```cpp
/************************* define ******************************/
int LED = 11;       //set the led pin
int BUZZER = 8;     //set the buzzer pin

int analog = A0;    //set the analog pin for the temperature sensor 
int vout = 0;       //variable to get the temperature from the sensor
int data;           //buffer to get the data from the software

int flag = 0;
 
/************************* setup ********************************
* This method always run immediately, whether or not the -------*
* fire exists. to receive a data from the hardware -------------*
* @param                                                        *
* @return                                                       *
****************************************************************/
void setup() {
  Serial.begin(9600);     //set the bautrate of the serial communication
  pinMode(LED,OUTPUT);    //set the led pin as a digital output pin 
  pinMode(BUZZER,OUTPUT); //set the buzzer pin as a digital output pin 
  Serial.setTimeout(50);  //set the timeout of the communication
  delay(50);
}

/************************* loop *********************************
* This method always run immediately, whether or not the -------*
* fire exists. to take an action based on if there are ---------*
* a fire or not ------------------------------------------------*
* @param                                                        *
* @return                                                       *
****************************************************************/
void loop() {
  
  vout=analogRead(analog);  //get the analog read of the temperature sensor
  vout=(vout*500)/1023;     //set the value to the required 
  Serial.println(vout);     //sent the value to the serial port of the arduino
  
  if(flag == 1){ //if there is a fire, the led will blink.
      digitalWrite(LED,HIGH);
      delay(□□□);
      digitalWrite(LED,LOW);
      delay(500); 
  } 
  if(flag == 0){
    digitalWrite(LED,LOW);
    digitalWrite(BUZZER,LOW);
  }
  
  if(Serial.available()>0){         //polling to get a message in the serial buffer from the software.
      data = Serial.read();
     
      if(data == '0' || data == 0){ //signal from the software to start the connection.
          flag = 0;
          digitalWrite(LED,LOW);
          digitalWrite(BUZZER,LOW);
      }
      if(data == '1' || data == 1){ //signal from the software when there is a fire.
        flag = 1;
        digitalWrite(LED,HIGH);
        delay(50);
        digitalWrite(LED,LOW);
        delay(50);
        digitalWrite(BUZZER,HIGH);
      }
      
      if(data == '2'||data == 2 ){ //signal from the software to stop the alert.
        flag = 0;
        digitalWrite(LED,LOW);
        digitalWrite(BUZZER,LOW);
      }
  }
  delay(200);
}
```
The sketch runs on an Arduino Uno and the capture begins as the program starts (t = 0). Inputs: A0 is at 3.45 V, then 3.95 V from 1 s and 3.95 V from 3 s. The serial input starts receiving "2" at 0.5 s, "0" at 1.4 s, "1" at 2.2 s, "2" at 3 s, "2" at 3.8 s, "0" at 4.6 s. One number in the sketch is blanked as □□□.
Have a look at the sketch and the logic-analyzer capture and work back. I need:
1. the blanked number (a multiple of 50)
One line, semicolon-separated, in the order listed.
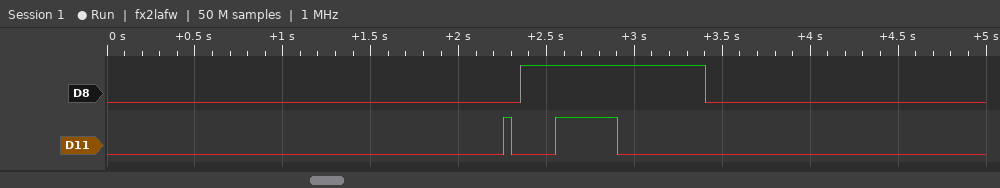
350
